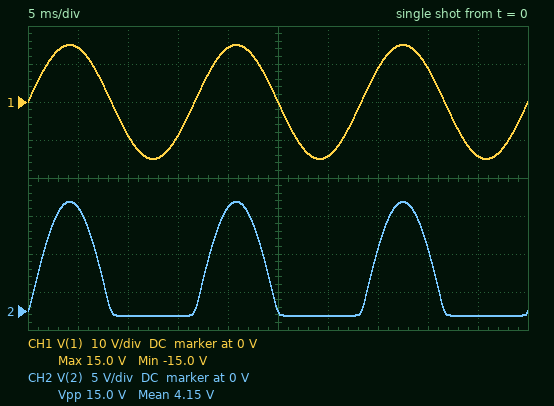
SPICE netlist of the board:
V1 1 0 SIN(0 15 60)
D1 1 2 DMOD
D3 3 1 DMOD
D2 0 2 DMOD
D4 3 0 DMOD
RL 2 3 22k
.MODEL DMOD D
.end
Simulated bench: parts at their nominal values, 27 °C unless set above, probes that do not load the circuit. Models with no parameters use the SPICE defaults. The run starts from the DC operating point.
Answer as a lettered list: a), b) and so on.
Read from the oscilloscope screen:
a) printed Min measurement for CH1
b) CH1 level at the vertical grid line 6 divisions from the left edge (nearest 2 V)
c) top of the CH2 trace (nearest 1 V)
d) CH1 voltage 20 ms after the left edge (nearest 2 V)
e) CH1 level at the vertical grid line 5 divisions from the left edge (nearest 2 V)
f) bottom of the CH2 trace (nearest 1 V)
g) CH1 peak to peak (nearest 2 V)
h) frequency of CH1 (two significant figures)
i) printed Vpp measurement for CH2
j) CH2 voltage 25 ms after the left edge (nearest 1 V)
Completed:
a) -15.0 V
b) -14 V
c) 14 V
d) 14 V
e) 0 V
f) -1 V
g) 30 V
h) 60 Hz
i) 15.0 V
j) 0 V
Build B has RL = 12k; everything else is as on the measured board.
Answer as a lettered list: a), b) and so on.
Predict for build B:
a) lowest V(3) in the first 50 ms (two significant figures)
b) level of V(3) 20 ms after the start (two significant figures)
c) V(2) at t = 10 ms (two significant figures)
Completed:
a) -14 V
b) 660 mV
c) -640 mV
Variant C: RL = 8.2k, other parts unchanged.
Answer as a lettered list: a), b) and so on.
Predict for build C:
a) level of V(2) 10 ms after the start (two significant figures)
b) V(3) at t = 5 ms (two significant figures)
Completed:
a) -650 mV
b) 670 mV
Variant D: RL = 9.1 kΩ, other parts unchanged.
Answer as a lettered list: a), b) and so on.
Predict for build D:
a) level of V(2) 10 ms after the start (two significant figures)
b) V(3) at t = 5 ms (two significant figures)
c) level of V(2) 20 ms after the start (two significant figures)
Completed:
a) -650 mV
b) 660 mV
c) 14 V
